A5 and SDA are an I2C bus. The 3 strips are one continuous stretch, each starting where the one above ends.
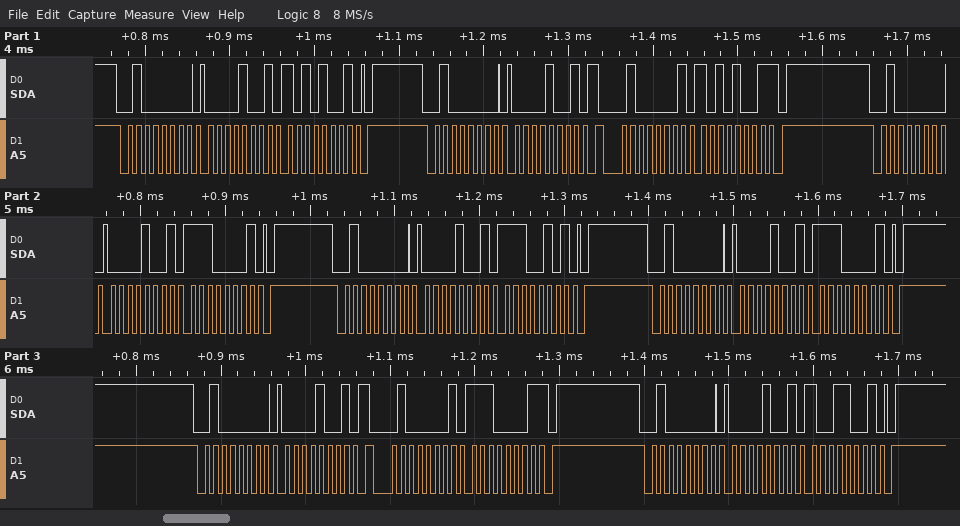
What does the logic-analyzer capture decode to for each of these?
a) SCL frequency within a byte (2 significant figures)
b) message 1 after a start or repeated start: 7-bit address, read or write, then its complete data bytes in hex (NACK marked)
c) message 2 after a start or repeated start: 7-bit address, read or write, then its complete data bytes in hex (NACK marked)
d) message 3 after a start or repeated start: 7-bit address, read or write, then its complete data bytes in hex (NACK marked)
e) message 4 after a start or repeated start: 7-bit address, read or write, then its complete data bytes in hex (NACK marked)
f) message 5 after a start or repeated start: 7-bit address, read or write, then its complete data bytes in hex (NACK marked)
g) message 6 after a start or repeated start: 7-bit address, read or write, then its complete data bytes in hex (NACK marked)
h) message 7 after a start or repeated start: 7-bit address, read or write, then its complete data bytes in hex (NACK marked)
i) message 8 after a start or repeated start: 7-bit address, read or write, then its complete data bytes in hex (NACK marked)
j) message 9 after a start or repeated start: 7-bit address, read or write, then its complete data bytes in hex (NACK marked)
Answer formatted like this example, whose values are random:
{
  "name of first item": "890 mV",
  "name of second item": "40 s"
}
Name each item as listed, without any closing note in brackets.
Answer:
{
  "SCL frequency within a byte": "100 kHz",
  "message 1 after a start or repeated start: 7-bit address, read or write, then its complete data bytes in hex": "0x20 write: 09 A9",
  "message 2 after a start or repeated start: 7-bit address, read or write, then its complete data bytes in hex": "0x20 write: 09",
  "message 3 after a start or repeated start: 7-bit address, read or write, then its complete data bytes in hex": "0x20 read: A9 NACK",
  "message 4 after a start or repeated start: 7-bit address, read or write, then its complete data bytes in hex": "0x20 write: 09 E1",
  "message 5 after a start or repeated start: 7-bit address, read or write, then its complete data bytes in hex": "0x20 write: 09 E5",
  "message 6 after a start or repeated start: 7-bit address, read or write, then its complete data bytes in hex": "0x20 write: 09 E1",
  "message 7 after a start or repeated start: 7-bit address, read or write, then its complete data bytes in hex": "0x20 write: 09",
  "message 8 after a start or repeated start: 7-bit address, read or write, then its complete data bytes in hex": "0x20 read: E1 NACK",
  "message 9 after a start or repeated start: 7-bit address, read or write, then its complete data bytes in hex": "0x20 write: 09 99"
}
